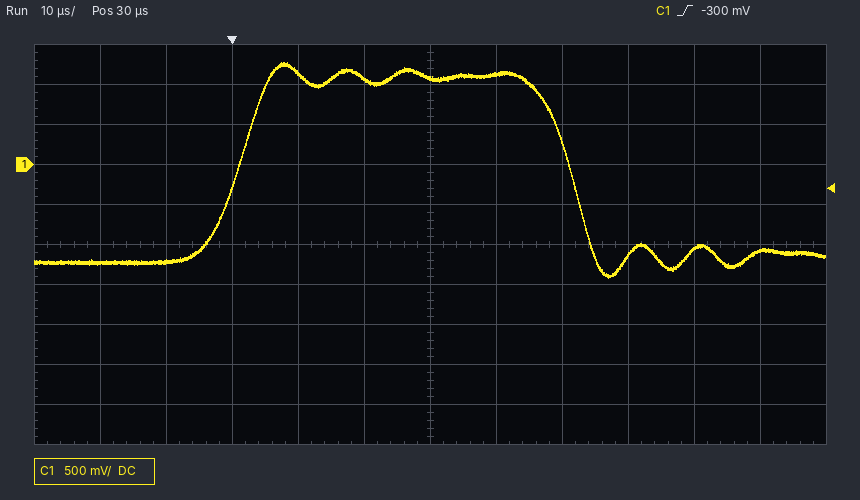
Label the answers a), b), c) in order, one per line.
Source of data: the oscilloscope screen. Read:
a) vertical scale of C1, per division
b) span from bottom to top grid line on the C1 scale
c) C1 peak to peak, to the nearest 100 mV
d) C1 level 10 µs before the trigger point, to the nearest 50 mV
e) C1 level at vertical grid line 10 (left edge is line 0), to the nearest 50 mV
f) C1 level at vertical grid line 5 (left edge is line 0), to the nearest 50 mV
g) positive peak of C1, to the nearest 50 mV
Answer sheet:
a) 500 mV
b) 5 V
c) 2.70 V
d) -1.20 V
e) -1.05 V
f) 1.05 V
g) 1.25 V
